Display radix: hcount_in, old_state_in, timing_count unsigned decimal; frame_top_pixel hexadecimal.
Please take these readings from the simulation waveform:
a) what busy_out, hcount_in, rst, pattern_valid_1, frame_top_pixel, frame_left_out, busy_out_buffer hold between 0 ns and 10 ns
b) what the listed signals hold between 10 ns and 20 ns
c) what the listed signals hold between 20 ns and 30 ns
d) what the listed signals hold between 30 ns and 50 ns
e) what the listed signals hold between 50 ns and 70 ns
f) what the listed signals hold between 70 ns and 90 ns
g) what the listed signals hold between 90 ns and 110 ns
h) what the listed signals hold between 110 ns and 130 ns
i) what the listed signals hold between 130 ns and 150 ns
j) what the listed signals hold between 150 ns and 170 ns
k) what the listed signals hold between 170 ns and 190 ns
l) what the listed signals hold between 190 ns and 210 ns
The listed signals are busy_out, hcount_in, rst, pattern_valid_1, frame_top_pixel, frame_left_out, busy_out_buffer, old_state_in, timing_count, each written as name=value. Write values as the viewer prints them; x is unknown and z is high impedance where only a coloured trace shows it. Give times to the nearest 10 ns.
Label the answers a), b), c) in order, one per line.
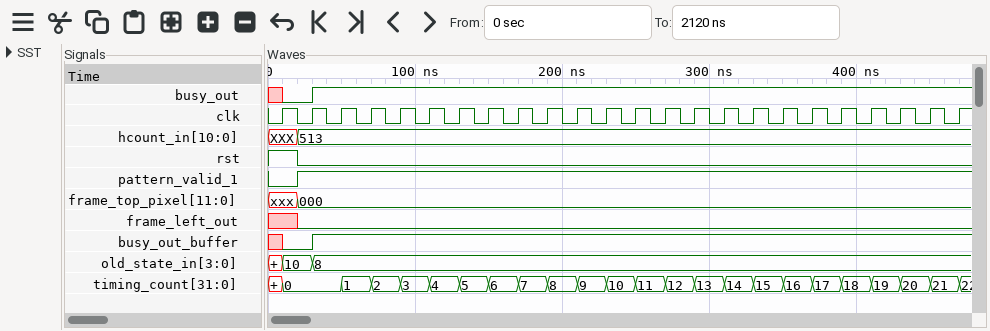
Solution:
a) busy_out=x, hcount_in=XXX, rst=1, pattern_valid_1=0, frame_top_pixel=xxx, frame_left_out=x, busy_out_buffer=x
b) busy_out=0, hcount_in=XXX, rst=1, pattern_valid_1=0, frame_top_pixel=xxx, frame_left_out=x, busy_out_buffer=0, old_state_in=10, timing_count=0
c) busy_out=0, hcount_in=513, rst=0, pattern_valid_1=1, frame_top_pixel=000, frame_left_out=0, busy_out_buffer=0, old_state_in=10, timing_count=0
d) busy_out=1, hcount_in=513, rst=0, pattern_valid_1=1, frame_top_pixel=000, frame_left_out=0, busy_out_buffer=1, old_state_in=8, timing_count=0
e) busy_out=1, hcount_in=513, rst=0, pattern_valid_1=1, frame_top_pixel=000, frame_left_out=0, busy_out_buffer=1, old_state_in=8, timing_count=1
f) busy_out=1, hcount_in=513, rst=0, pattern_valid_1=1, frame_top_pixel=000, frame_left_out=0, busy_out_buffer=1, old_state_in=8, timing_count=2
g) busy_out=1, hcount_in=513, rst=0, pattern_valid_1=1, frame_top_pixel=000, frame_left_out=0, busy_out_buffer=1, old_state_in=8, timing_count=3
h) busy_out=1, hcount_in=513, rst=0, pattern_valid_1=1, frame_top_pixel=000, frame_left_out=0, busy_out_buffer=1, old_state_in=8, timing_count=4
i) busy_out=1, hcount_in=513, rst=0, pattern_valid_1=1, frame_top_pixel=000, frame_left_out=0, busy_out_buffer=1, old_state_in=8, timing_count=5
j) busy_out=1, hcount_in=513, rst=0, pattern_valid_1=1, frame_top_pixel=000, frame_left_out=0, busy_out_buffer=1, old_state_in=8, timing_count=6
k) busy_out=1, hcount_in=513, rst=0, pattern_valid_1=1, frame_top_pixel=000, frame_left_out=0, busy_out_buffer=1, old_state_in=8, timing_count=7
l) busy_out=1, hcount_in=513, rst=0, pattern_valid_1=1, frame_top_pixel=000, frame_left_out=0, busy_out_buffer=1, old_state_in=8, timing_count=8
